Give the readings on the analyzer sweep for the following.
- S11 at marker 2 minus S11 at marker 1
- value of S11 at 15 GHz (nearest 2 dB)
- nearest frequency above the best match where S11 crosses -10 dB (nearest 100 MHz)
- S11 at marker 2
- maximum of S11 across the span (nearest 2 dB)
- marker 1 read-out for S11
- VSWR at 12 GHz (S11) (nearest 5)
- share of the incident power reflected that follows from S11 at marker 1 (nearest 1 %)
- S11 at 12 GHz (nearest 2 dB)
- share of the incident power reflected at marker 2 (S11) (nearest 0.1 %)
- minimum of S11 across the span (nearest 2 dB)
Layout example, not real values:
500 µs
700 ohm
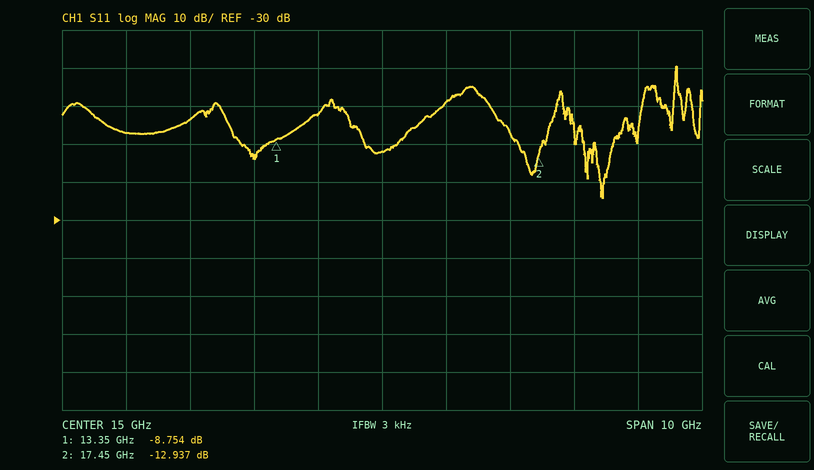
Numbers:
-4.183 dB
-12 dB
18.6 GHz
-12.937 dB
10 dB
-8.754 dB
5
13 %
-4 dB
5.1 %
-24 dB
